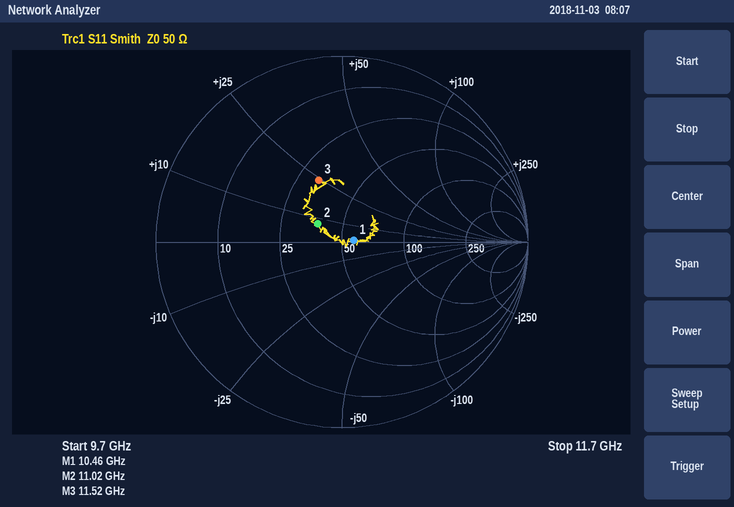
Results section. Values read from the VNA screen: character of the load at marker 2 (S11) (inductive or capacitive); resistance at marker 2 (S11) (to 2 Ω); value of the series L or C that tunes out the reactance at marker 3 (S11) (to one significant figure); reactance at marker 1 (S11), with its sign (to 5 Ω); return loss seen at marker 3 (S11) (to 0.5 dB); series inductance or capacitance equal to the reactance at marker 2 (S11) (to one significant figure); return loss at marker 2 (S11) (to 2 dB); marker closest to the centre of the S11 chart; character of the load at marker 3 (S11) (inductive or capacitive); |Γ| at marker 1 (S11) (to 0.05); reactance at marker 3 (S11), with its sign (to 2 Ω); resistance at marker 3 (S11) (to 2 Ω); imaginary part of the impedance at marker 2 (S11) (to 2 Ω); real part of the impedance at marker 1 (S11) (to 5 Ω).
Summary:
inductive
38 Ω
600 fF
0 Ω
9.0 dB
100 pH
16 dB
marker 1
inductive
0.05
+24 Ω
32 Ω
+8 Ω
55 Ω
